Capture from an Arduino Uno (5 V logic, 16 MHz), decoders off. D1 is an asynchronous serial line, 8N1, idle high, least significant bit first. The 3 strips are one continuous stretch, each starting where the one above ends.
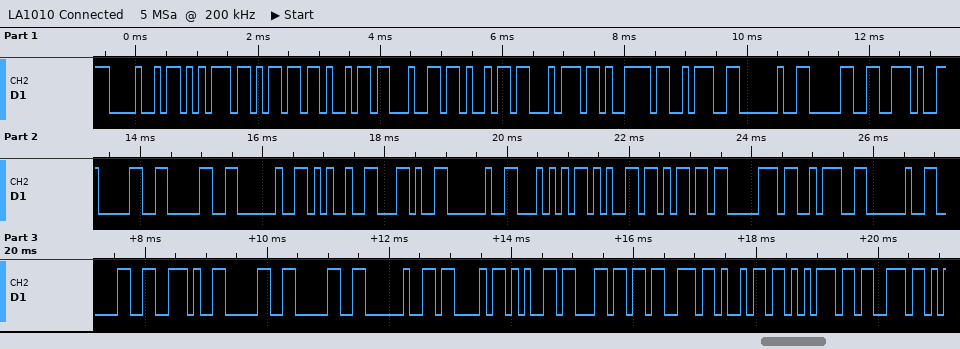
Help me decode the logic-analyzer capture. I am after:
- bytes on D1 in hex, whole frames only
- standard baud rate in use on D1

48 75 6D 69 64 69 74 79 3A 20 30 2E 30 30 20 25 2C 20 54 65 6D 70 3A 20 30 2E 30 30 20 43 65 6C 73 69 75 73
9600 baud
